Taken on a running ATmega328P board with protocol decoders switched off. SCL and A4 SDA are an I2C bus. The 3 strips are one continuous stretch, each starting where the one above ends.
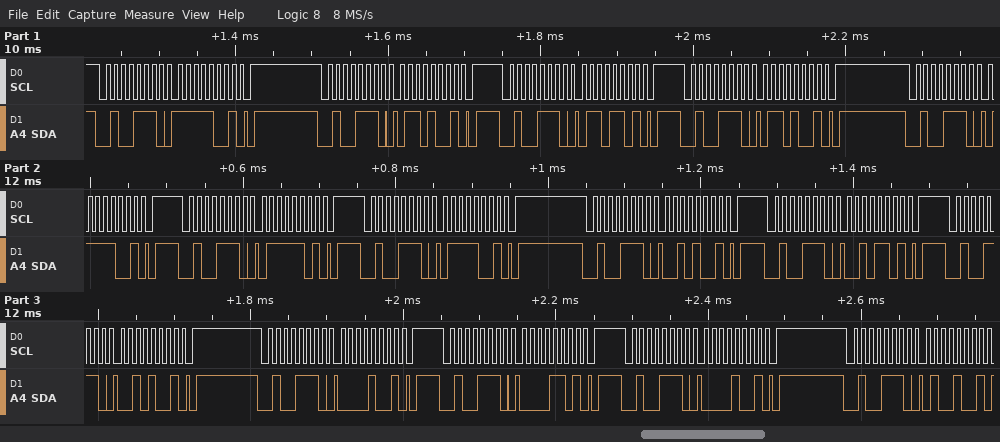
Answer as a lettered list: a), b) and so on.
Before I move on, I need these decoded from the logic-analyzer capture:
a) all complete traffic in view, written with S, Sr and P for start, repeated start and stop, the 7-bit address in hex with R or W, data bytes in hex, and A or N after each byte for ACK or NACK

a) S 27W A F9 A P S 27W A 69 A P S 27W A 6D A P S 27W A 69 A P S 27W A 79 A P S 27W A 7D A P S 27W A 79 A P S 27W A 29 A P S 27W A 2D A P S 27W A 29 A P S 27W A 09 A P S 27W A 0D A P S 27W A 09 A P S 27W A 49 A
